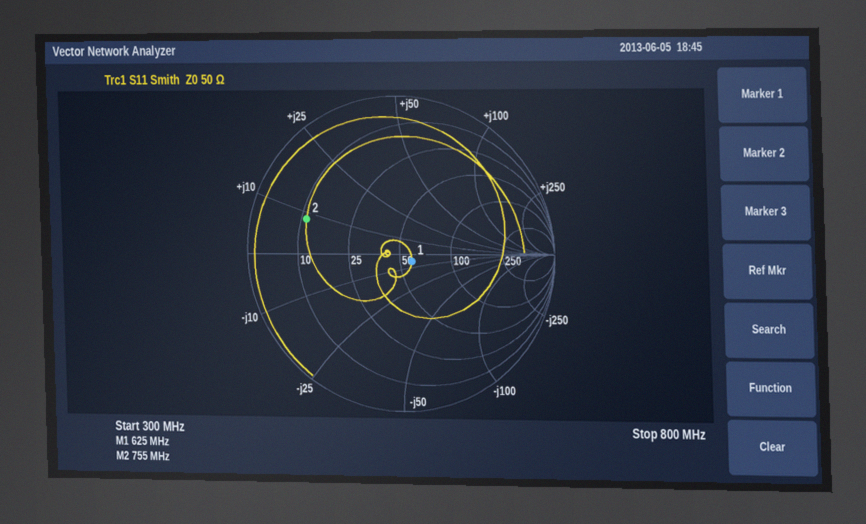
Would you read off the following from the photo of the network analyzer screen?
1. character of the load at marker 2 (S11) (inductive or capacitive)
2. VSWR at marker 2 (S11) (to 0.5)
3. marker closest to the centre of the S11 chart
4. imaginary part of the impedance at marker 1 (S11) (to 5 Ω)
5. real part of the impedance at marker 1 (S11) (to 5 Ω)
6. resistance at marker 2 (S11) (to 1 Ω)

inductive
4.5
marker 1
-5 Ω
60 Ω
11 Ω
